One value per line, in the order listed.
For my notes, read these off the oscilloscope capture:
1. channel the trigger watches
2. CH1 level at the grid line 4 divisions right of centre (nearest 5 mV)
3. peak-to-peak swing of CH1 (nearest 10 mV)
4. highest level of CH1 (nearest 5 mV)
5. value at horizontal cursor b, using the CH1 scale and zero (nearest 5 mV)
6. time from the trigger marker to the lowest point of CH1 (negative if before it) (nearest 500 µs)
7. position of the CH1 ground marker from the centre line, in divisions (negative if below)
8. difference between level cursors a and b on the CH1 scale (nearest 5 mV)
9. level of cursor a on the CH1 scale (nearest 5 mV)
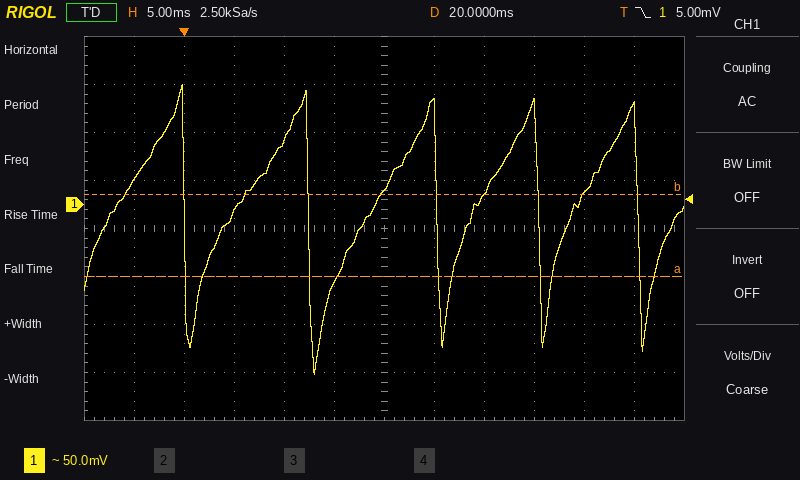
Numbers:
CH1
10 mV
300 mV
125 mV
10 mV
+13.0 ms
+0.5 div
85 mV
-75 mV
